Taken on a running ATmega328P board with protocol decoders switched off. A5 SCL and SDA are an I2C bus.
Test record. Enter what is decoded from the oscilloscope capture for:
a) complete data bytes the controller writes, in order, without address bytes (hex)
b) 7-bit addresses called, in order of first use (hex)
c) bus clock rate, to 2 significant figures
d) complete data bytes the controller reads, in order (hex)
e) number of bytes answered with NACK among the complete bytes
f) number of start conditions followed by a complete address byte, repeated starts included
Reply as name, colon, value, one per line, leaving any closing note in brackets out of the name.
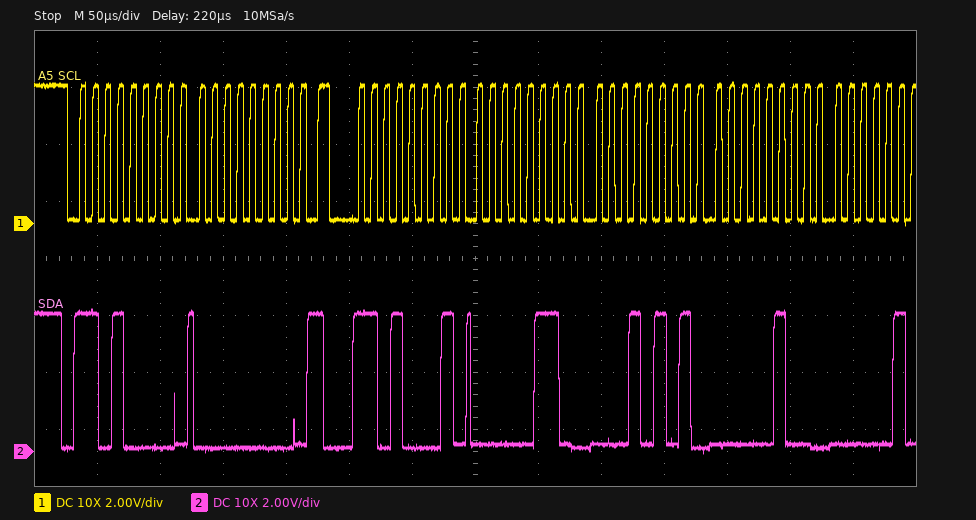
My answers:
complete data bytes the controller writes, in order, without address bytes: 00
7-bit addresses called, in order of first use: 0x68
bus clock rate, to 2 significant figures: 100 kHz
complete data bytes the controller reads, in order: 06 15 04
number of bytes answered with NACK among the complete bytes: 0
number of start conditions followed by a complete address byte, repeated starts included: 2
